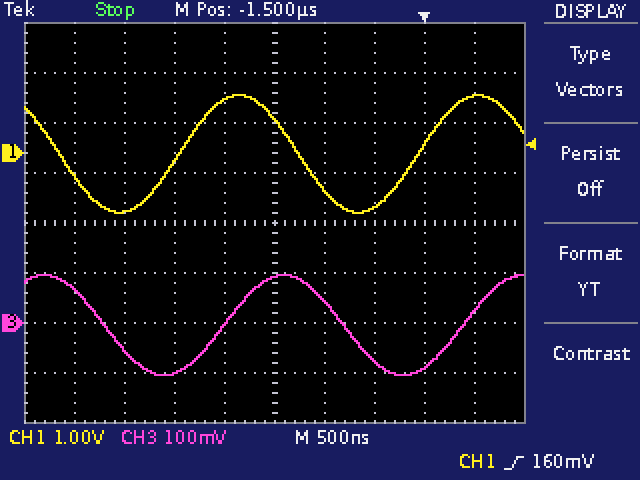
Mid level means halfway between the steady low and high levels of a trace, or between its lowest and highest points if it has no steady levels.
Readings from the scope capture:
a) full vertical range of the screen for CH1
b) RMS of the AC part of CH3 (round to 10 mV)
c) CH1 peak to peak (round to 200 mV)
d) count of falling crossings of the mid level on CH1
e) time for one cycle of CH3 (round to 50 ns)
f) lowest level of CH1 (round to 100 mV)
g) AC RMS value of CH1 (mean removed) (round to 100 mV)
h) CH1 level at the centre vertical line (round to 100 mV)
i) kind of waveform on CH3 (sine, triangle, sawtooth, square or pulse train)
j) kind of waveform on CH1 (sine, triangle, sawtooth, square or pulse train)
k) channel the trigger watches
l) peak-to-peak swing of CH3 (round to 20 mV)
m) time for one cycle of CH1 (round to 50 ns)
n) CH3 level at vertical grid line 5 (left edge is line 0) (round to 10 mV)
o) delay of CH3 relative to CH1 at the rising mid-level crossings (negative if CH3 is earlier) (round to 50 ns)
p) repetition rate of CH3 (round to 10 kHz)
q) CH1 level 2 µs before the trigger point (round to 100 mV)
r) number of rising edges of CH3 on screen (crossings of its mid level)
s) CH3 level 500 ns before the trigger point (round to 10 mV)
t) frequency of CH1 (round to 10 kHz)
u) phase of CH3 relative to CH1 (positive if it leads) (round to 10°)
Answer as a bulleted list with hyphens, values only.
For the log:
- 8 V
- 70 mV
- 2.4 V
- 2
- 2.40 µs
- -1.2 V
- 800 mV
- 700 mV
- sine
- sine
- CH1
- 200 mV
- 2.40 µs
- 90 mV
- +450 ns
- 420 kHz
- 1.1 V
- 2
- -80 mV
- 420 kHz
- -70°
